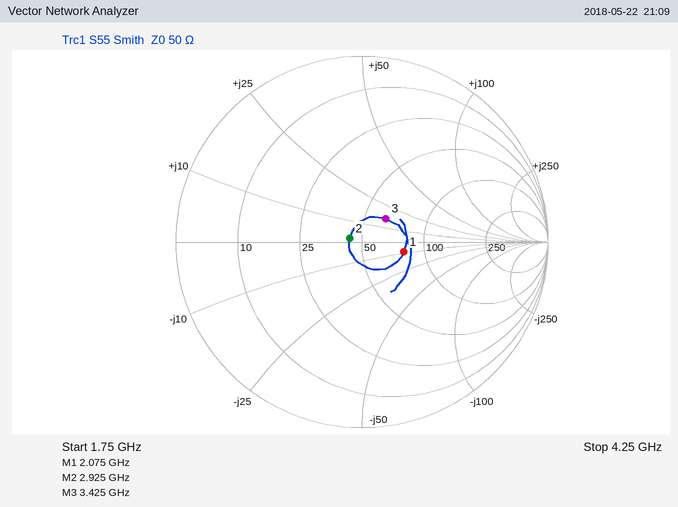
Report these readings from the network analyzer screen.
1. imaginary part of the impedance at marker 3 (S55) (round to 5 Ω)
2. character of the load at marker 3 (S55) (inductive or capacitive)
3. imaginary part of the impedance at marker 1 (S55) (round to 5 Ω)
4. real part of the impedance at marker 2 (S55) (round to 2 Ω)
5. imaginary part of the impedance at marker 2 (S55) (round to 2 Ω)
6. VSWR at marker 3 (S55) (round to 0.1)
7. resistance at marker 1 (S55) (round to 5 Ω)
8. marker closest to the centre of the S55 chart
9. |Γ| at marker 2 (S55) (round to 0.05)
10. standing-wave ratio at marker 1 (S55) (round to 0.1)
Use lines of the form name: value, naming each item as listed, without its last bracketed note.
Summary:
imaginary part of the impedance at marker 3 (S55): +15 Ω
character of the load at marker 3 (S55): inductive
imaginary part of the impedance at marker 1 (S55): -10 Ω
real part of the impedance at marker 2 (S55): 44 Ω
imaginary part of the impedance at marker 2 (S55): +2 Ω
VSWR at marker 3 (S55): 1.4
resistance at marker 1 (S55): 80 Ω
marker closest to the centre of the S55 chart: marker 2
|Γ| at marker 2 (S55): 0.05
standing-wave ratio at marker 1 (S55): 1.6
